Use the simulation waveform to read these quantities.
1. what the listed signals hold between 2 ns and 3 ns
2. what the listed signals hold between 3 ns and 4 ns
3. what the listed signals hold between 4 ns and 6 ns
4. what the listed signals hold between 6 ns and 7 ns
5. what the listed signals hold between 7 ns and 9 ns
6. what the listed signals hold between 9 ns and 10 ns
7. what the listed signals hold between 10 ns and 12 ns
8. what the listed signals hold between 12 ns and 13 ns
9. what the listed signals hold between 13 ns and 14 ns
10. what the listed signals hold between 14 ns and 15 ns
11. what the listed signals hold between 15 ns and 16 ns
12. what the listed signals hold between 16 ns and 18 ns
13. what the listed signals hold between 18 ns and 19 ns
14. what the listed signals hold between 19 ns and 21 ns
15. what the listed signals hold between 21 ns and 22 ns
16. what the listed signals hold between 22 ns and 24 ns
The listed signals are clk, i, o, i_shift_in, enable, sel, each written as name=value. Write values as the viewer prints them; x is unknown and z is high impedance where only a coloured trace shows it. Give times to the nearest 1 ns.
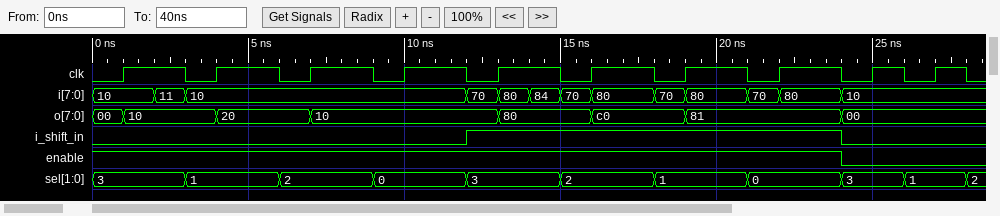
clk=1, i=11, o=10, i_shift_in=0, enable=1, sel=3
clk=0, i=10, o=10, i_shift_in=0, enable=1, sel=1
clk=1, i=10, o=20, i_shift_in=0, enable=1, sel=1
clk=0, i=10, o=20, i_shift_in=0, enable=1, sel=2
clk=1, i=10, o=10, i_shift_in=0, enable=1, sel=2
clk=0, i=10, o=10, i_shift_in=0, enable=1, sel=0
clk=1, i=10, o=10, i_shift_in=0, enable=1, sel=0
clk=0, i=70, o=10, i_shift_in=1, enable=1, sel=3
clk=1, i=80, o=80, i_shift_in=1, enable=1, sel=3
clk=1, i=84, o=80, i_shift_in=1, enable=1, sel=3
clk=0, i=70, o=80, i_shift_in=1, enable=1, sel=2
clk=1, i=80, o=c0, i_shift_in=1, enable=1, sel=2
clk=0, i=70, o=c0, i_shift_in=1, enable=1, sel=1
clk=1, i=80, o=81, i_shift_in=1, enable=1, sel=1
clk=0, i=70, o=81, i_shift_in=1, enable=1, sel=0
clk=1, i=80, o=81, i_shift_in=1, enable=1, sel=0
